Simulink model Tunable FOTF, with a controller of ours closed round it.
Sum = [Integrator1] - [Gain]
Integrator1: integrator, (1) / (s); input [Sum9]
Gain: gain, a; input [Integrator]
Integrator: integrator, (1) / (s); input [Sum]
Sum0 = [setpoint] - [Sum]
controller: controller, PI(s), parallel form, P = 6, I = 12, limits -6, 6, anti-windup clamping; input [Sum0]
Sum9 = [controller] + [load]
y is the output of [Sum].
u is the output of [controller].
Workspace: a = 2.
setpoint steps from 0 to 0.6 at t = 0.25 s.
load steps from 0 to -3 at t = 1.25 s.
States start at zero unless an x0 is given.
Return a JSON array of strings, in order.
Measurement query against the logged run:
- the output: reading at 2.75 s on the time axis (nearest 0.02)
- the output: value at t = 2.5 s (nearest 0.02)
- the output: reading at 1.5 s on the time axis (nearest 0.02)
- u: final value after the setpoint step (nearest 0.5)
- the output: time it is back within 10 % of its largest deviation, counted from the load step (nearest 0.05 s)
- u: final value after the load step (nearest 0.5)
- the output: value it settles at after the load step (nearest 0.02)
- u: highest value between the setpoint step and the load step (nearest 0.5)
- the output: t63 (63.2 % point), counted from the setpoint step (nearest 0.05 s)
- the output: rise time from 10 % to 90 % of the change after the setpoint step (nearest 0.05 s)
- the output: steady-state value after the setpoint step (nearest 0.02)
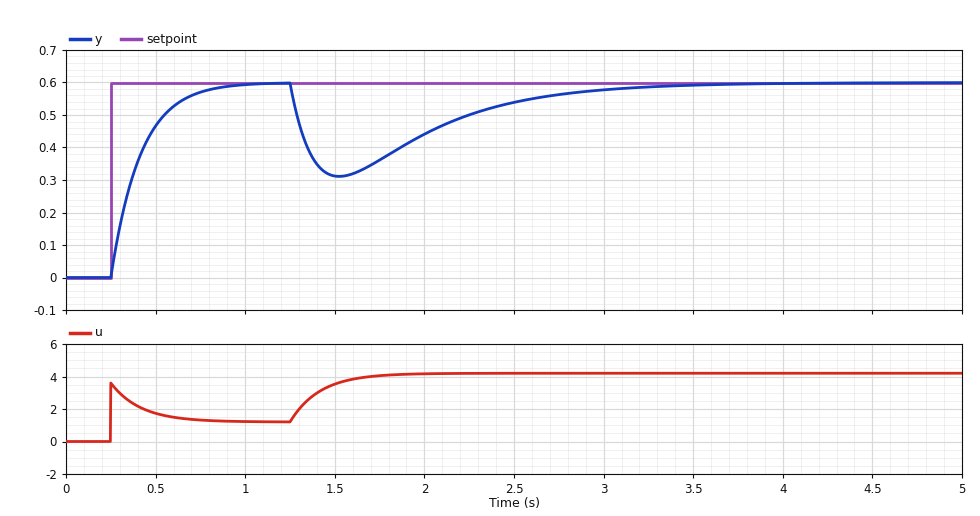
["0.56", "0.54", "0.32", "1.0", "1.65 s", "4.0", "0.60", "3.5", "0.15 s", "0.35 s", "0.60"]
